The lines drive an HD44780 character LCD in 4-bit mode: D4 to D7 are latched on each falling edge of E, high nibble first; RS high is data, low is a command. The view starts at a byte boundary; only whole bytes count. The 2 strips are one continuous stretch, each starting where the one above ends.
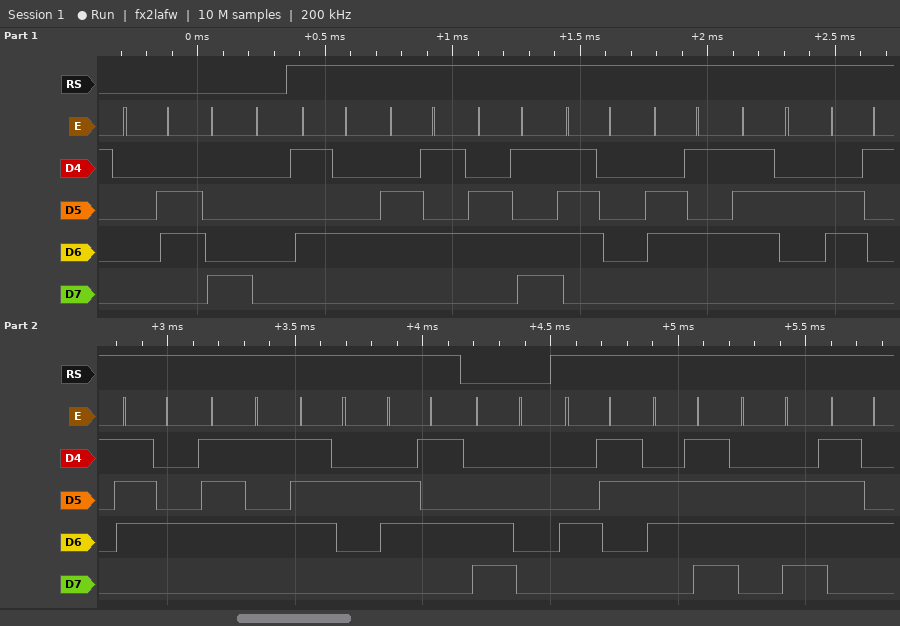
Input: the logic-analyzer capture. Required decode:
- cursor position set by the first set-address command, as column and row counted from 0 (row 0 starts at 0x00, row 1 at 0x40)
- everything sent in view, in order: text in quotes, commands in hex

column 0, row 0
0x06 0x80 "Temperature" 0xC0 "Cont"
